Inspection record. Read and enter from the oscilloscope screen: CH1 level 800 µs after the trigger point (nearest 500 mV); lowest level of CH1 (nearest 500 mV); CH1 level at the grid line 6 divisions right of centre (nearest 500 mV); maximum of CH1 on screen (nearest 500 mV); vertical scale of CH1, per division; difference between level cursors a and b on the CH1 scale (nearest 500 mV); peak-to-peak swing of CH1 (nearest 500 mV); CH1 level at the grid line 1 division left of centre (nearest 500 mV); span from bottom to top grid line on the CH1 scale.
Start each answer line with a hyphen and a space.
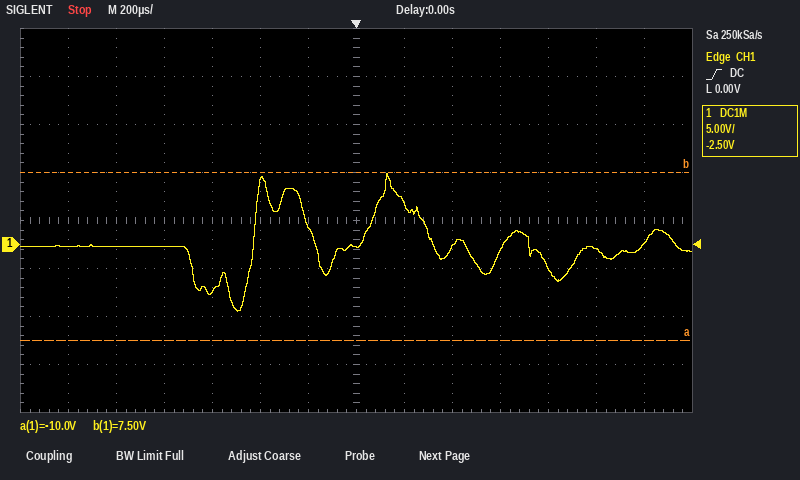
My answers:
- -2.5 V
- -7.0 V
- 0.0 V
- 7.5 V
- 5 V
- 17.5 V
- 14.5 V
- 2.0 V
- 40 V
